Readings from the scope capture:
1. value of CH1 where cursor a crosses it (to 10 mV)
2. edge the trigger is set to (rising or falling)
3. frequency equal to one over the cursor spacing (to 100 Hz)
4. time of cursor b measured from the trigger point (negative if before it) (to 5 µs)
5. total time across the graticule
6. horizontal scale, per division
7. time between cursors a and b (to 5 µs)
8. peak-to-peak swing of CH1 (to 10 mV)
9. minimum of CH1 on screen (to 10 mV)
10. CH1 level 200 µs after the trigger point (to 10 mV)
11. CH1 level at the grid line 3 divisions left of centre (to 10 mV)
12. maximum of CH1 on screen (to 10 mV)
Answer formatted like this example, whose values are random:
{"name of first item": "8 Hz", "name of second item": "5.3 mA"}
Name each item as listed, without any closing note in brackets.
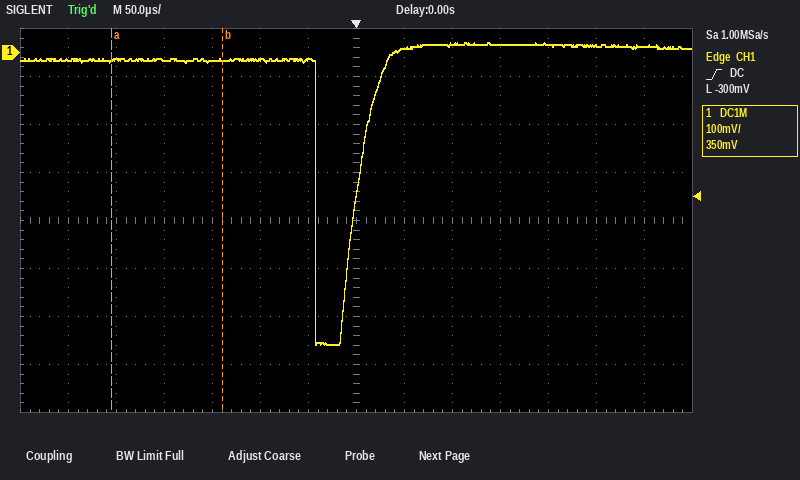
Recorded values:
{"value of CH1 where cursor a crosses it": "-20 mV", "edge the trigger is set to": "rising", "frequency equal to one over the cursor spacing": "8.7 kHz", "time of cursor b measured from the trigger point (negative if before it)": "-140 µs", "total time across the graticule": "700 µs", "horizontal scale, per division": "50 µs", "time between cursors a and b": "115 µs", "peak-to-peak swing of CH1": "630 mV", "minimum of CH1 on screen": "-610 mV", "CH1 level 200 µs after the trigger point": "20 mV", "CH1 level at the grid line 3 divisions left of centre": "-20 mV", "maximum of CH1 on screen": "20 mV"}
